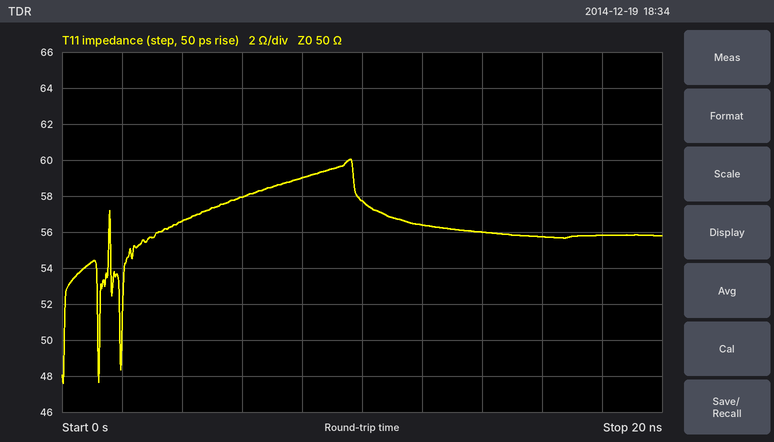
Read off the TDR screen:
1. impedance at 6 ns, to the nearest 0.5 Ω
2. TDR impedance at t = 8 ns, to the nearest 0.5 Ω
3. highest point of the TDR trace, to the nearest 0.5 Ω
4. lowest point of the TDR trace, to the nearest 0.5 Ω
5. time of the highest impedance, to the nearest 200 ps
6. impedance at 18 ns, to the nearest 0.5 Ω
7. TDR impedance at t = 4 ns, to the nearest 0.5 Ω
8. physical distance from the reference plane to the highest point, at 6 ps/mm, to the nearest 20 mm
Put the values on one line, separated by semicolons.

58.0 Ω; 59.0 Ω; 60.0 Ω; 47.5 Ω; 9.6 ns; 56.0 Ω; 56.5 Ω; 800 mm
